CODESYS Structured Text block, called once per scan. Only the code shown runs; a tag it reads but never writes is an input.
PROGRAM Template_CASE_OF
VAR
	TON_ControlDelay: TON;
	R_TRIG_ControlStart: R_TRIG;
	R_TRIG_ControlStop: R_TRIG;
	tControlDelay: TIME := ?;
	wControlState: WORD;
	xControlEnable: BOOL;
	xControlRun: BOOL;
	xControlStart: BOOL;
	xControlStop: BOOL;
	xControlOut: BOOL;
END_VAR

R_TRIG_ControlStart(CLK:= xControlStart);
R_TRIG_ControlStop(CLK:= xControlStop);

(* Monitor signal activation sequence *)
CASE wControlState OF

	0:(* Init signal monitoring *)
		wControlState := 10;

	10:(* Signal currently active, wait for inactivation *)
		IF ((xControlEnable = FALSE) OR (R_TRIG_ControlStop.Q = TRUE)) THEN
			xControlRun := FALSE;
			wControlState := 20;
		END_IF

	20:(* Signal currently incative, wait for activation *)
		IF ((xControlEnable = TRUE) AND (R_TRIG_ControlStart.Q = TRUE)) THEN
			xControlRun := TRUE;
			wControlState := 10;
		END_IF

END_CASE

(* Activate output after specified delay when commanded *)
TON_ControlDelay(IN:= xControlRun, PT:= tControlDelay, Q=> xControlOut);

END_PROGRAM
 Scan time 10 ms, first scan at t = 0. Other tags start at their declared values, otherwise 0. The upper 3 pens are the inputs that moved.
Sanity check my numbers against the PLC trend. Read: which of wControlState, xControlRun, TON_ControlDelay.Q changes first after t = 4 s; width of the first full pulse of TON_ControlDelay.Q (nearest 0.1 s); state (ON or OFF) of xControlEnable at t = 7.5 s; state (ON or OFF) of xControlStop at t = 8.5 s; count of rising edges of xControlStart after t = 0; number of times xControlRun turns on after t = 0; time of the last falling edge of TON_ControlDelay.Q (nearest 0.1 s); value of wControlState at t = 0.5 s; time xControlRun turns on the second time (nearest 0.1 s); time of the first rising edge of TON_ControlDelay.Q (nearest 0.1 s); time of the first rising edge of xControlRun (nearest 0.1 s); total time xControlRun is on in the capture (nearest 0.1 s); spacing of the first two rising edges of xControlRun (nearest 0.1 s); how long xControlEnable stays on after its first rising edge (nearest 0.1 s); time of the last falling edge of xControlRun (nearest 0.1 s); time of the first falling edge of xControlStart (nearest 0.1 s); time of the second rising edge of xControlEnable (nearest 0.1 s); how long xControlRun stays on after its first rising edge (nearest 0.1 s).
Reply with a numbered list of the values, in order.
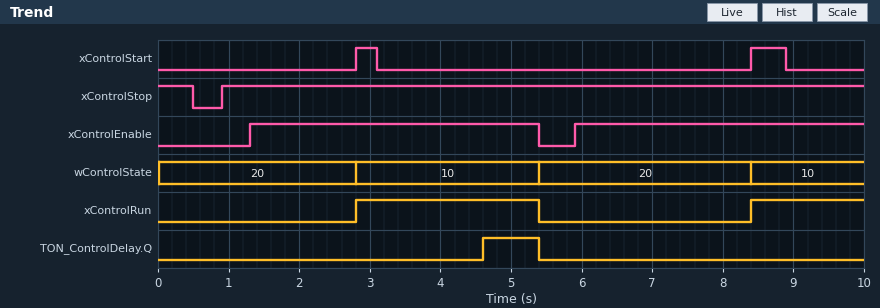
1. TON_ControlDelay.Q
2. 0.8 s
3. ON
4. ON
5. 2
6. 2
7. 5.4 s
8. 20
9. 8.4 s
10. 4.6 s
11. 2.8 s
12. 4.2 s
13. 5.6 s
14. 4.1 s
15. 5.4 s
16. 3.1 s
17. 5.9 s
18. 2.6 s
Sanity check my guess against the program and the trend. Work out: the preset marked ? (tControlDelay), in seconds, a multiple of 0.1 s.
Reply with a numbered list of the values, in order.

1. 1.8 s
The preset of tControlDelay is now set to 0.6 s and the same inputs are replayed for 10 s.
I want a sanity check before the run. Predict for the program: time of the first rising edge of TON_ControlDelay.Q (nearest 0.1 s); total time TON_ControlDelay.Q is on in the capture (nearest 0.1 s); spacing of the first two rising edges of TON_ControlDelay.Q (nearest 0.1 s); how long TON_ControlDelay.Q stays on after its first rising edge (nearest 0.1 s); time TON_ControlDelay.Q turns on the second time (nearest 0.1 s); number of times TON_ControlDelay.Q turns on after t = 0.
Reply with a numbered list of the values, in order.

1. 3.4 s
2. 3.0 s
3. 5.6 s
4. 2.0 s
5. 9.0 s
6. 2
